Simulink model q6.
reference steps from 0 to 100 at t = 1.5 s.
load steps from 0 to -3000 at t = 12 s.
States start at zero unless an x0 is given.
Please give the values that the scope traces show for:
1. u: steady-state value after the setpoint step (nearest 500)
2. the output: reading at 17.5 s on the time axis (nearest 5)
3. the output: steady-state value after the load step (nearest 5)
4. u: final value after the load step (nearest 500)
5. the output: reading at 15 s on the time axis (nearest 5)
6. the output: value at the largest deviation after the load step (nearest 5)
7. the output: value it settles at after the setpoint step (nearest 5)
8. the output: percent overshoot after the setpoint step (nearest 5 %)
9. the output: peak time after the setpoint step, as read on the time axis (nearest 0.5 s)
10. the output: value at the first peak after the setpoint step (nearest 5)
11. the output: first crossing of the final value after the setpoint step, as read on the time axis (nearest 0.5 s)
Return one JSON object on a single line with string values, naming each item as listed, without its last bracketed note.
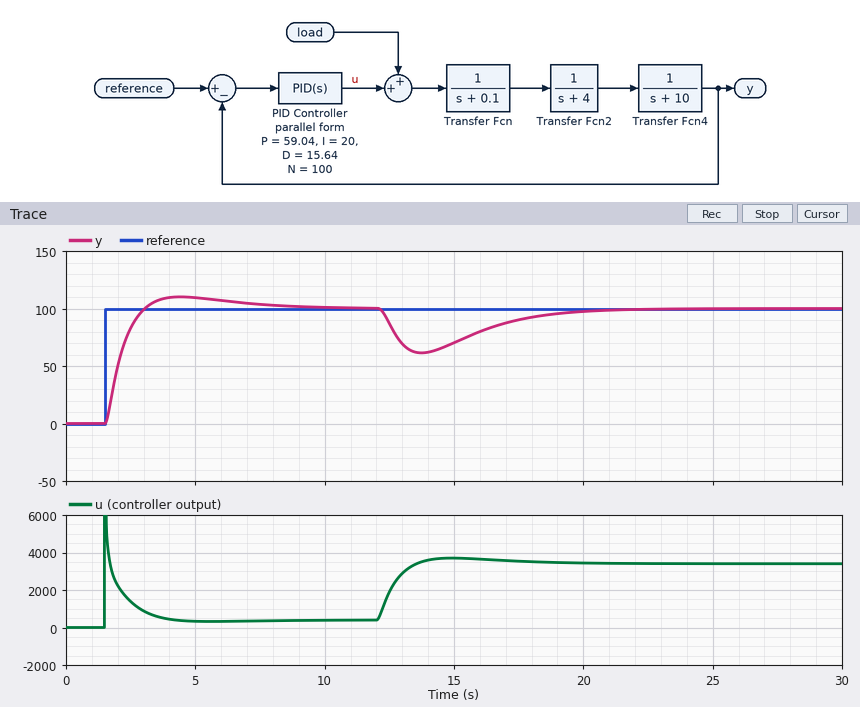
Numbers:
{"u: steady-state value after the setpoint step": "500", "the output: reading at 17.5 s on the time axis": "90", "the output: steady-state value after the load step": "100", "u: final value after the load step": "3500", "the output: reading at 15 s on the time axis": "70", "the output: value at the largest deviation after the load step": "60", "the output: value it settles at after the setpoint step": "100", "the output: percent overshoot after the setpoint step": "10 %", "the output: peak time after the setpoint step, as read on the time axis": "4.5 s", "the output: value at the first peak after the setpoint step": "110", "the output: first crossing of the final value after the setpoint step, as read on the time axis": "3.0 s"}
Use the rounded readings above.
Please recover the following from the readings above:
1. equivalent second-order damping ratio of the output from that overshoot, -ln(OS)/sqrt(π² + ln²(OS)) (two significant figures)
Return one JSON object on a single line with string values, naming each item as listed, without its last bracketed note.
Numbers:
{"equivalent second-order damping ratio of the output from that overshoot, -ln(OS)/sqrt(π² + ln²(OS))": "0.59"}
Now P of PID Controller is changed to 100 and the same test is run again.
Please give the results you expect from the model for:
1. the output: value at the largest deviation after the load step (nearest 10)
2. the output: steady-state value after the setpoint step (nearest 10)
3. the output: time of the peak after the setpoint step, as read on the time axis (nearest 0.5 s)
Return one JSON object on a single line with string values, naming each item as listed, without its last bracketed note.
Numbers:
{"the output: value at the largest deviation after the load step": "70", "the output: steady-state value after the setpoint step": "100", "the output: time of the peak after the setpoint step, as read on the time axis": "3.0 s"}
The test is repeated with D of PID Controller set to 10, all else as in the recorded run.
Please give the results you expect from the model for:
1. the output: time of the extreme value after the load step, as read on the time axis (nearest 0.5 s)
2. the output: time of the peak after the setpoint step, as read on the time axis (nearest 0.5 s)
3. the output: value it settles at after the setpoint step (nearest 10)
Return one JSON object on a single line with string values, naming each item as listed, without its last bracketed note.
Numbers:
{"the output: time of the extreme value after the load step, as read on the time axis": "13.5 s", "the output: time of the peak after the setpoint step, as read on the time axis": "4.0 s", "the output: value it settles at after the setpoint step": "100"}
